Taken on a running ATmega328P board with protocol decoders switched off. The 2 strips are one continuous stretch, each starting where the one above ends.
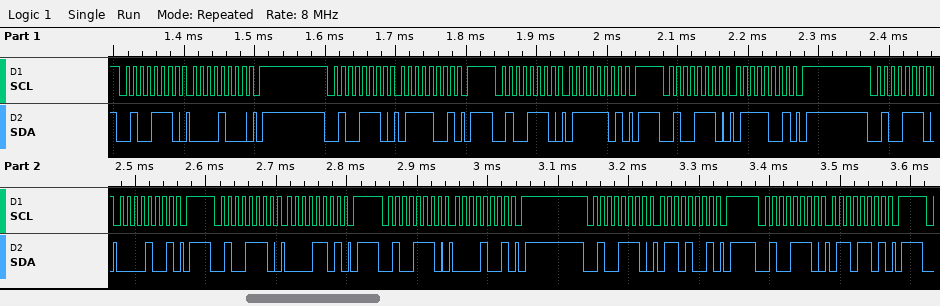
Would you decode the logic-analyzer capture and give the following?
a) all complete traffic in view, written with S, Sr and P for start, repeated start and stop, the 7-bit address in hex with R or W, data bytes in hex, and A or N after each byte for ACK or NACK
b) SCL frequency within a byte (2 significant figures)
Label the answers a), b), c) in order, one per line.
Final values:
a) S 27W A 08 A P S 27W A 79 A P S 27W A 7D A P S 27W A 79 A P S 27W A 09 A P S 27W A 0D A P S 27W A 09 A P S 27W A 69 A P S 27W A 6D A P
b) 100 kHz
